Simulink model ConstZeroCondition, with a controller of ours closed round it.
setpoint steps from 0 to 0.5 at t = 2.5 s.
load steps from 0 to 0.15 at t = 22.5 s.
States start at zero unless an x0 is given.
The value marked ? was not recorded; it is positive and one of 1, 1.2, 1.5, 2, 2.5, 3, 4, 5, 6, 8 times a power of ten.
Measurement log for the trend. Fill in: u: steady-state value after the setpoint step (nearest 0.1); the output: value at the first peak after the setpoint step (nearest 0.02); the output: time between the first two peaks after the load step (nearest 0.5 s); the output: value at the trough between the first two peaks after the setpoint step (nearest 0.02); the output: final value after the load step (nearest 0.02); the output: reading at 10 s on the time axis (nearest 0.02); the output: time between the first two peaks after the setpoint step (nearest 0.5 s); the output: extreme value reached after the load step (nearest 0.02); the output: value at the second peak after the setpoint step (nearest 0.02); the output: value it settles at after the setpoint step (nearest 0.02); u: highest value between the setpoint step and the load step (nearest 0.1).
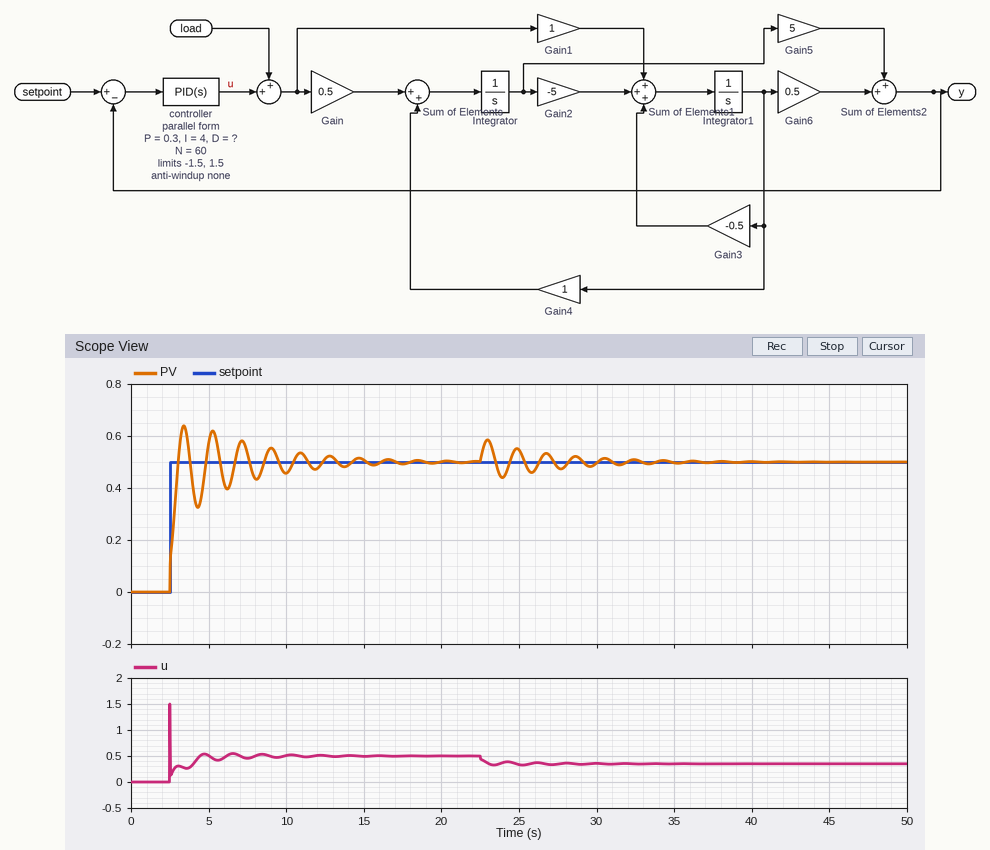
0.5
0.64
2.0 s
0.32
0.50
0.46
2.0 s
0.58
0.62
0.50
1.5
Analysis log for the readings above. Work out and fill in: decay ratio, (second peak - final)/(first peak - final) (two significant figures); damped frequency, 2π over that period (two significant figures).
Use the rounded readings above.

0.86
3.1 rad/s
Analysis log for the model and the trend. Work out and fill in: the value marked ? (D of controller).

0.2
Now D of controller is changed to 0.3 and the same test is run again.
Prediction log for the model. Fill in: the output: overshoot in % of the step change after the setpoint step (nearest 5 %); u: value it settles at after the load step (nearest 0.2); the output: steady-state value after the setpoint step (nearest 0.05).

25 %
0.4
0.50
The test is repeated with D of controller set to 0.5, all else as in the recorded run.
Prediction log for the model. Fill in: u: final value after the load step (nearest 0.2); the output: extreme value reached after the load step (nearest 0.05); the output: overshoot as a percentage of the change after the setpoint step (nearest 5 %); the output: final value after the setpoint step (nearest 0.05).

0.4
0.55
25 %
0.50
